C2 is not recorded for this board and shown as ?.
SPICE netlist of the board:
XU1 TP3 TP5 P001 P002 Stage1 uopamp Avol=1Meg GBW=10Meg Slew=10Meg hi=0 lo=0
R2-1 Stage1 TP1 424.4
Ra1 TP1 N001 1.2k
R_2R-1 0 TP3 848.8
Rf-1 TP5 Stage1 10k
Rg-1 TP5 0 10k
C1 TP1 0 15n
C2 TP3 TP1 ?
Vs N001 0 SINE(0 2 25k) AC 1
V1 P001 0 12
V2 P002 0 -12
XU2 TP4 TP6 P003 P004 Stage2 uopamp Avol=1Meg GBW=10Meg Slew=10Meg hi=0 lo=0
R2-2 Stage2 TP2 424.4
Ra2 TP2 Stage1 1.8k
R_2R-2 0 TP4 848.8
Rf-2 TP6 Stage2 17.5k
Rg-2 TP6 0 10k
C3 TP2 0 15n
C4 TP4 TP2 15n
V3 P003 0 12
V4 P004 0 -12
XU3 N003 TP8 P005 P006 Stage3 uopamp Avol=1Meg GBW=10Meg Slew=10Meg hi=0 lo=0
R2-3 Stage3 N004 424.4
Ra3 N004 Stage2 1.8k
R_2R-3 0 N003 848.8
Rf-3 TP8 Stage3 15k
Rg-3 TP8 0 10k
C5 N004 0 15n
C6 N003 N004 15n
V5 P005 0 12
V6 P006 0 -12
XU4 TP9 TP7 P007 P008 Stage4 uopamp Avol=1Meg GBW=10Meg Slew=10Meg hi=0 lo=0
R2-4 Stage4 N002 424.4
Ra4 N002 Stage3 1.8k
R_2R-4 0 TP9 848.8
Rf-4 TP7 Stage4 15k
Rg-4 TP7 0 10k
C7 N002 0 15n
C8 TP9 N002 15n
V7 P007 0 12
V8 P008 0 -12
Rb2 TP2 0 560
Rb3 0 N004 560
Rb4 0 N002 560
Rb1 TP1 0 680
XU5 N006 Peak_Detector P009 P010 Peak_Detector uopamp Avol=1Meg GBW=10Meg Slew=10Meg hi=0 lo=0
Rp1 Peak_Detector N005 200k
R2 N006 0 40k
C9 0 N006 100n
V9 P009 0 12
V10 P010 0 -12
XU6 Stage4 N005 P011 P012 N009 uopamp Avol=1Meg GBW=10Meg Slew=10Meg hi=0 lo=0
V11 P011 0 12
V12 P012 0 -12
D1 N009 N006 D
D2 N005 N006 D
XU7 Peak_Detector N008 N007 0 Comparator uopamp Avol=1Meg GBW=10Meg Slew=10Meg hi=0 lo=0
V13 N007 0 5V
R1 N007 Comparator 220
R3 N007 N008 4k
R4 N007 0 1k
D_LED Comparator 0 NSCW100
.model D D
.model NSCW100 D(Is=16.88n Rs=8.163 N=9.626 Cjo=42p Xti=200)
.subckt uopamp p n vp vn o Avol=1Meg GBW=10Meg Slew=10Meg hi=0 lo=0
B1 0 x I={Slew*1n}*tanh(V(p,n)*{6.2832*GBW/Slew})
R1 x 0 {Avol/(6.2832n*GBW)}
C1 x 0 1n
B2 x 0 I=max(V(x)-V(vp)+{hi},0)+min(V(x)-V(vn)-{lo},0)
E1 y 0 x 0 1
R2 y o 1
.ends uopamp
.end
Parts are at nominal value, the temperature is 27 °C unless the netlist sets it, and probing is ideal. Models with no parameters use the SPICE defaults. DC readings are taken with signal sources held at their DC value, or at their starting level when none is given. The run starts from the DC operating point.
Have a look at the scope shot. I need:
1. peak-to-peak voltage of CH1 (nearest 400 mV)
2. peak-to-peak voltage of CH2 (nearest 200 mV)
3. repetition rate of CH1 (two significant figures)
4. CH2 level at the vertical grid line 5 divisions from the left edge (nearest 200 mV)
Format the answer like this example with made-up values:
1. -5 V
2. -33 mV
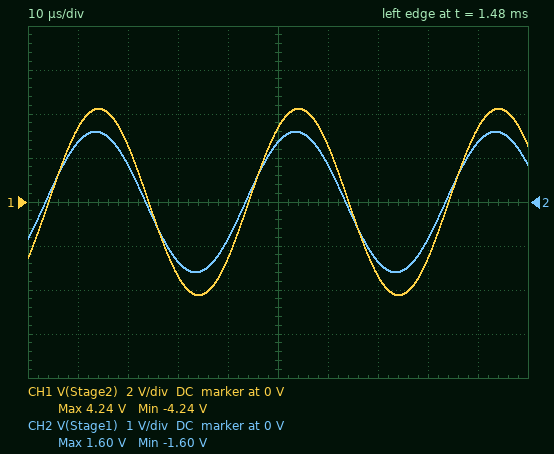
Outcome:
1. 8.4 V
2. 3.2 V
3. 25 kHz
4. 1.4 V
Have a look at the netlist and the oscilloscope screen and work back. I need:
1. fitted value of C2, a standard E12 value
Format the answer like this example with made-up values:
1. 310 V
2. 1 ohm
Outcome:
1. 27 nF
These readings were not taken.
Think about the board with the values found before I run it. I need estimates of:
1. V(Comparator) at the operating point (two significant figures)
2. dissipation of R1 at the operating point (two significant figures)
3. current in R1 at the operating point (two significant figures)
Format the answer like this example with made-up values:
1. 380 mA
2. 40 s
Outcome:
1. 13 mV
2. 110 mW
3. 23 mA
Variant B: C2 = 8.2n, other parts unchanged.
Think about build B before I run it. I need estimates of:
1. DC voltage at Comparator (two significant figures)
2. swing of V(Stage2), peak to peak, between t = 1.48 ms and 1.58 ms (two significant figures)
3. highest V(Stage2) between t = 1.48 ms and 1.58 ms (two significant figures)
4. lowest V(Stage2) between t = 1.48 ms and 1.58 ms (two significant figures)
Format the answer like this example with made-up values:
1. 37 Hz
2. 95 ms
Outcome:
1. 13 mV
2. 4.7 V
3. 2.3 V
4. -2.3 V
